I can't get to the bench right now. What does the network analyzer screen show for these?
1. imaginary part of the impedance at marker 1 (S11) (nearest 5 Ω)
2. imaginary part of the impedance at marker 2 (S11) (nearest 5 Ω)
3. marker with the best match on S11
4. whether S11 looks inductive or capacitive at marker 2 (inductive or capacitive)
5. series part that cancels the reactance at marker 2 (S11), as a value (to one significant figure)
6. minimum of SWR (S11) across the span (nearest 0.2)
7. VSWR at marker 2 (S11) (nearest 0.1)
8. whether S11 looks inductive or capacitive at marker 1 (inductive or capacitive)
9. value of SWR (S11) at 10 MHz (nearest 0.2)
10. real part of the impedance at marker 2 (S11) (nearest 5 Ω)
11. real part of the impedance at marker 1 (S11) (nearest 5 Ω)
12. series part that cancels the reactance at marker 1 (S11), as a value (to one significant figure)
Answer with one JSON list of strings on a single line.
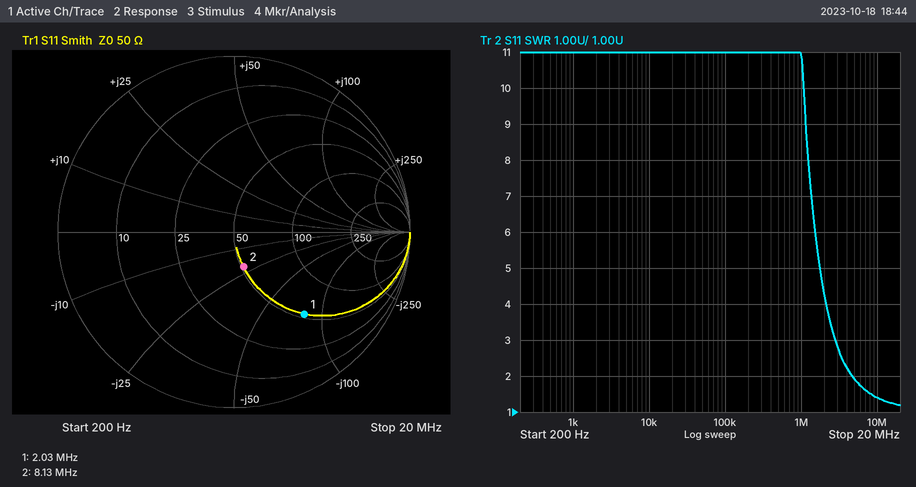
["-80 Ω", "-20 Ω", "marker 2", "capacitive", "400 nH", "1.2", "1.5", "capacitive", "1.4", "50 Ω", "55 Ω", "6 µH"]
